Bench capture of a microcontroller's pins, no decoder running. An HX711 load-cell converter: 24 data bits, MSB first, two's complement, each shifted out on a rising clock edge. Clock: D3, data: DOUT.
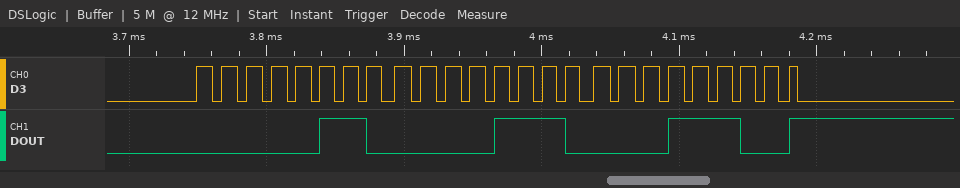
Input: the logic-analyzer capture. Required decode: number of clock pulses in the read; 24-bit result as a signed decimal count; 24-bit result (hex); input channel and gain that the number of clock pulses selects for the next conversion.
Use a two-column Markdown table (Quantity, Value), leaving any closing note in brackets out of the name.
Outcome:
| Quantity | Value |
|---|---|
| number of clock pulses in the read | 25 |
| 24-bit result as a signed decimal count | 396828 |
| 24-bit result | 0x060E1C |
| input channel and gain that the number of clock pulses selects for the next conversion | channel A, gain 128 |
